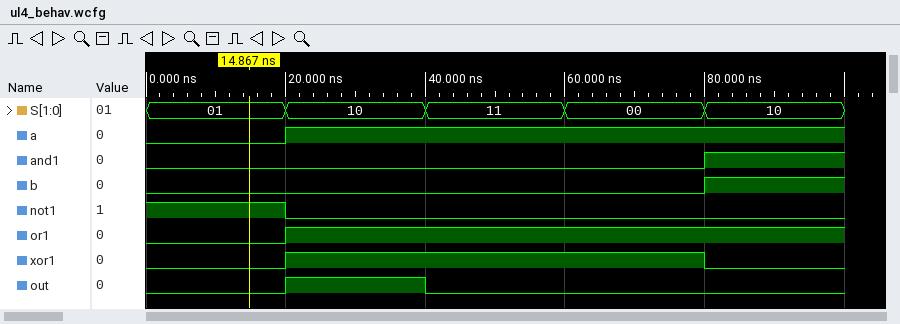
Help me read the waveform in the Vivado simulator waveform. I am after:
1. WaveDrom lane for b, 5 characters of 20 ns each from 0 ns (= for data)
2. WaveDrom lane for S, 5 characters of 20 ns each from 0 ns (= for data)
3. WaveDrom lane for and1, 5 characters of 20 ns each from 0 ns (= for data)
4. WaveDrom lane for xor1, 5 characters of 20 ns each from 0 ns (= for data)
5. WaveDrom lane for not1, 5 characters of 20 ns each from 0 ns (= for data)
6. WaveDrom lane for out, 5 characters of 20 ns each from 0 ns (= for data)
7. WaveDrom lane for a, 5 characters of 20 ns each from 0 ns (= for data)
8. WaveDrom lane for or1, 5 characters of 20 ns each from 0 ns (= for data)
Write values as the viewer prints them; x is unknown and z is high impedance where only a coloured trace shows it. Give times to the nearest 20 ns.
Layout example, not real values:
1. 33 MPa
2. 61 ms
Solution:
1. {name: 'b', wave: '0...1'}
2. {name: 'S', wave: '=====', data: '01 10 11 00 10'}
3. {name: 'and1', wave: '0...1'}
4. {name: 'xor1', wave: '01..0'}
5. {name: 'not1', wave: '10...'}
6. {name: 'out', wave: '010..'}
7. {name: 'a', wave: '01...'}
8. {name: 'or1', wave: '01...'}
